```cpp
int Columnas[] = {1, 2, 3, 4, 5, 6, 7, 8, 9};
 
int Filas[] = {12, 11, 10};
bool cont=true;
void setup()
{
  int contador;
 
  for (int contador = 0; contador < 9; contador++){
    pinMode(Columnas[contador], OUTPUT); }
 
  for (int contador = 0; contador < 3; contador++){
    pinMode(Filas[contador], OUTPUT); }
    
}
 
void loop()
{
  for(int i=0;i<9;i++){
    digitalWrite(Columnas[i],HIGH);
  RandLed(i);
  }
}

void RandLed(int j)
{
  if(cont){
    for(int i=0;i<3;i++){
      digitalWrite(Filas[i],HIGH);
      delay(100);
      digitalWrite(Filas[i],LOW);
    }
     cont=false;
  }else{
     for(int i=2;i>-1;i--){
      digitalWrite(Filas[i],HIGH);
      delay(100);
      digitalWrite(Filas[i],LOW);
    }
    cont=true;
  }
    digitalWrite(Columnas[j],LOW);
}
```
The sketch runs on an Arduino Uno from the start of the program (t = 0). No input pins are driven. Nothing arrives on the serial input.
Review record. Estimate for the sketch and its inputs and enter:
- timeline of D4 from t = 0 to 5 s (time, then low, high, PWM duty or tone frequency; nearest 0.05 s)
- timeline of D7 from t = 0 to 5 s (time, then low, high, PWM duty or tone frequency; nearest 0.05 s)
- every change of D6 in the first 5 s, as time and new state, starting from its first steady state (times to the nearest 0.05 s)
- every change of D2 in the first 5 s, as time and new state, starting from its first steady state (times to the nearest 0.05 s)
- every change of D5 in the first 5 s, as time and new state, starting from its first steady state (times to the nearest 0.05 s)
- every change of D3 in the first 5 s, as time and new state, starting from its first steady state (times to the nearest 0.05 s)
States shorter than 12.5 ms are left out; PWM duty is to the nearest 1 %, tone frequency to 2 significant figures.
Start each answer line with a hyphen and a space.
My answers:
- 0 s low; 0.9 s high; 1.2 s low; 3.6 s high; 3.9 s low
- 0 s low; 1.8 s high; 2.1 s low; 4.5 s high; 4.8 s low
- 0 s low; 1.5 s high; 1.8 s low; 4.2 s high; 4.5 s low
- 0 s low; 0.3 s high; 0.6 s low; 3 s high; 3.3 s low
- 0 s low; 1.2 s high; 1.5 s low; 3.9 s high; 4.2 s low
- 0 s low; 0.6 s high; 0.9 s low; 3.3 s high; 3.6 s low
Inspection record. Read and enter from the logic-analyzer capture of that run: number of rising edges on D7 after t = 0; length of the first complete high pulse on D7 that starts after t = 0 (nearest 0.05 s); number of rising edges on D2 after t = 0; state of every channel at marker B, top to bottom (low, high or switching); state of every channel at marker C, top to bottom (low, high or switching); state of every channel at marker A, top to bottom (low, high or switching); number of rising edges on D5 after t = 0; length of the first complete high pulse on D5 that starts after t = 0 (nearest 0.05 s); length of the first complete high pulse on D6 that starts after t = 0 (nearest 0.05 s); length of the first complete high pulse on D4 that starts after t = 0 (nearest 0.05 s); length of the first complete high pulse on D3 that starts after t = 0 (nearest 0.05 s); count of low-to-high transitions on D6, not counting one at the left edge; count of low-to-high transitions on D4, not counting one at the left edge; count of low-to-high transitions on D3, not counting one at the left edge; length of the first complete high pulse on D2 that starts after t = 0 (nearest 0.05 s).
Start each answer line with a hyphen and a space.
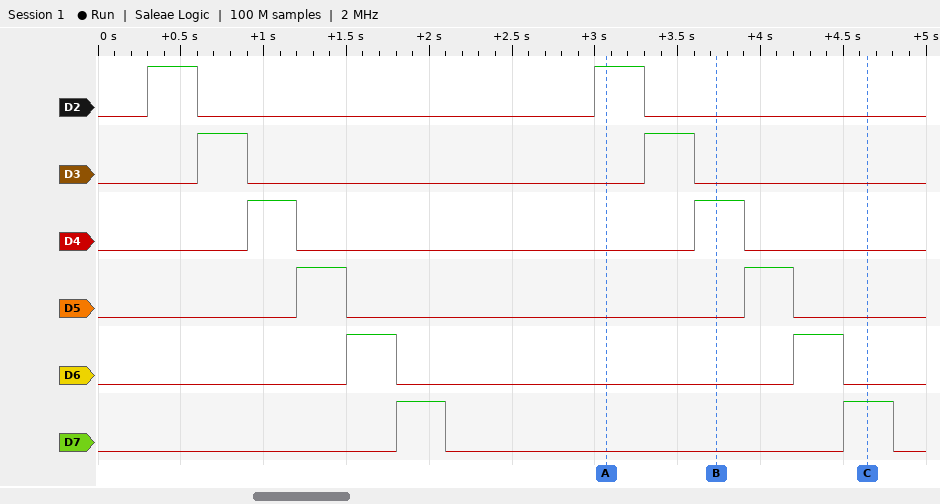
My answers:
- 2
- 0.30 s
- 2
- D2 low, D3 low, D4 high, D5 low, D6 low, D7 low
- D2 low, D3 low, D4 low, D5 low, D6 low, D7 high
- D2 high, D3 low, D4 low, D5 low, D6 low, D7 low
- 2
- 0.30 s
- 0.30 s
- 0.30 s
- 0.30 s
- 2
- 2
- 2
- 0.30 s
